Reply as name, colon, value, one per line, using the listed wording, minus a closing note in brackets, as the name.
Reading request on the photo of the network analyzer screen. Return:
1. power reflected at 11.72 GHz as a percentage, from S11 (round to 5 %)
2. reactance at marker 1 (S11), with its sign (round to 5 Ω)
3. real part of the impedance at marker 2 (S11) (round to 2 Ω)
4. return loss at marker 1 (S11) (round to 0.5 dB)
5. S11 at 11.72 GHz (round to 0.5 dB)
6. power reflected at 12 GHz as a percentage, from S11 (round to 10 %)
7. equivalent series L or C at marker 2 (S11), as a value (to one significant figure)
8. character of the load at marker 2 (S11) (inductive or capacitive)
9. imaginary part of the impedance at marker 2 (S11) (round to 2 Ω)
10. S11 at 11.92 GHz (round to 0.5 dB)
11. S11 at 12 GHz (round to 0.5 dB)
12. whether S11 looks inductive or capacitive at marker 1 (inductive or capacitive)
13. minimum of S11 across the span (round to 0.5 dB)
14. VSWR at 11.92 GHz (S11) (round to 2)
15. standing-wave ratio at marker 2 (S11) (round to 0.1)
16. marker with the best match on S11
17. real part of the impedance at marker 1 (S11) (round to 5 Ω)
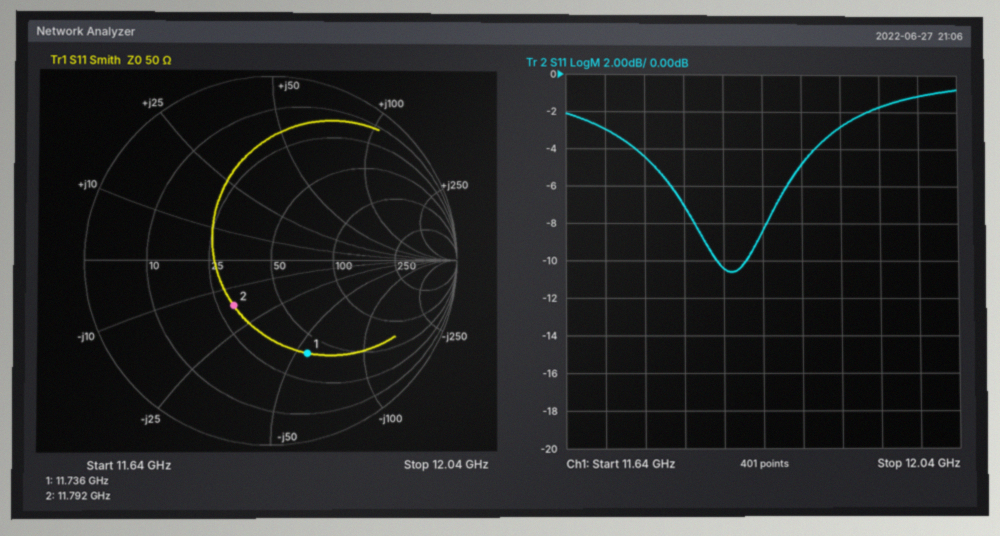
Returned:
power reflected at 11.72 GHz as a percentage, from S11: 35 %
reactance at marker 1 (S11), with its sign: -55 Ω
real part of the impedance at marker 2 (S11): 30 Ω
return loss at marker 1 (S11): 5.5 dB
S11 at 11.72 GHz: -4.5 dB
power reflected at 12 GHz as a percentage, from S11: 80 %
equivalent series L or C at marker 2 (S11), as a value: 800 fF
character of the load at marker 2 (S11): capacitive
imaginary part of the impedance at marker 2 (S11): -16 Ω
S11 at 11.92 GHz: -3.0 dB
S11 at 12 GHz: -1.0 dB
whether S11 looks inductive or capacitive at marker 1: capacitive
minimum of S11 across the span: -10.5 dB
VSWR at 11.92 GHz (S11): 6
standing-wave ratio at marker 2 (S11): 1.9
marker with the best match on S11: marker 2
real part of the impedance at marker 1 (S11): 40 Ω
